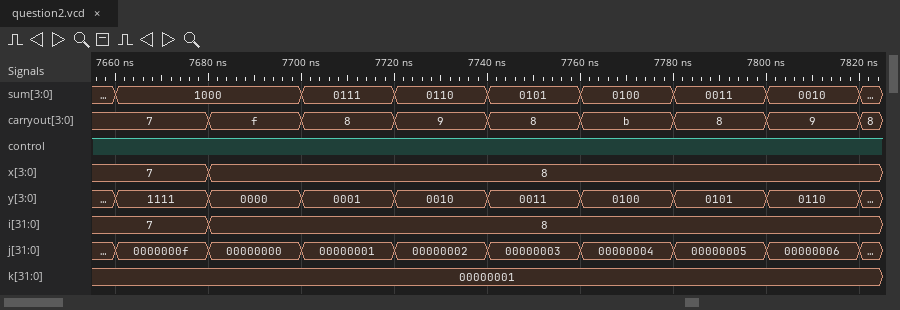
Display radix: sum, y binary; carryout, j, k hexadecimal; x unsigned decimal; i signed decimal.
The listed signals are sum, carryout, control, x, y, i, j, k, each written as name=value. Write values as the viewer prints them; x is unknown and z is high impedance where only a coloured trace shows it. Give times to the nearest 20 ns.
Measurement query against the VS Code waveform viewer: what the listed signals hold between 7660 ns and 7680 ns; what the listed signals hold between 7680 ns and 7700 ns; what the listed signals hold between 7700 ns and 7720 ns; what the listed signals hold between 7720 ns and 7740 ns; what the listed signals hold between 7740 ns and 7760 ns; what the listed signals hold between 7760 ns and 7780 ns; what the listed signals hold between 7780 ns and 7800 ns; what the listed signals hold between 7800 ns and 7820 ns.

sum=1000, carryout=7, control=1, x=7, y=1111, i=7, j=0000000f, k=00000001
sum=1000, carryout=f, control=1, x=8, y=0000, i=8, j=00000000, k=00000001
sum=0111, carryout=8, control=1, x=8, y=0001, i=8, j=00000001, k=00000001
sum=0110, carryout=9, control=1, x=8, y=0010, i=8, j=00000002, k=00000001
sum=0101, carryout=8, control=1, x=8, y=0011, i=8, j=00000003, k=00000001
sum=0100, carryout=b, control=1, x=8, y=0100, i=8, j=00000004, k=00000001
sum=0011, carryout=8, control=1, x=8, y=0101, i=8, j=00000005, k=00000001
sum=0010, carryout=9, control=1, x=8, y=0110, i=8, j=00000006, k=00000001
